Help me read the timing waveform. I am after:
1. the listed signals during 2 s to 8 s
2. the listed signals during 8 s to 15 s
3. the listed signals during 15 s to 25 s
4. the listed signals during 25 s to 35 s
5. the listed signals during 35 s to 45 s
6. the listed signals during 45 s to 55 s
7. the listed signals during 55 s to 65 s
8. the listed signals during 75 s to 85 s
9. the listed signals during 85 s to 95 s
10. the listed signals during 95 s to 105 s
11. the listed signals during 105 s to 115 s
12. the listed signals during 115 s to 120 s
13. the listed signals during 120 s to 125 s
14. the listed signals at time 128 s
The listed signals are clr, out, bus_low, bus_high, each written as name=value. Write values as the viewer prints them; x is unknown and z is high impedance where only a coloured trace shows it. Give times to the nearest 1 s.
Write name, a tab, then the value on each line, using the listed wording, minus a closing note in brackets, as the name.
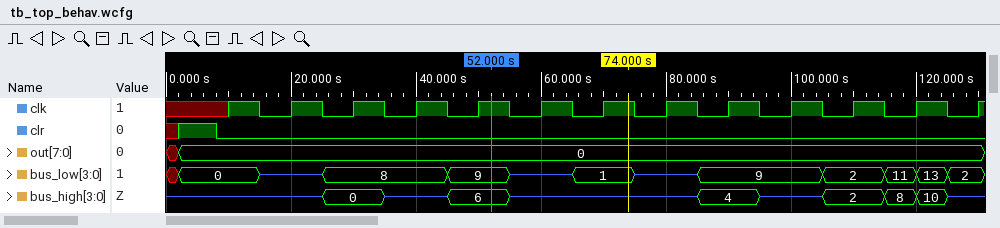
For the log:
the listed signals during 2 s to 8 s	clr=1, out=0, bus_low=0, bus_high=z
the listed signals during 8 s to 15 s	clr=0, out=0, bus_low=0, bus_high=z
the listed signals during 15 s to 25 s	clr=0, out=0, bus_low=z, bus_high=z
the listed signals during 25 s to 35 s	clr=0, out=0, bus_low=8, bus_high=0
the listed signals during 35 s to 45 s	clr=0, out=0, bus_low=8, bus_high=z
the listed signals during 45 s to 55 s	clr=0, out=0, bus_low=9, bus_high=6
the listed signals during 55 s to 65 s	clr=0, out=0, bus_low=z, bus_high=z
the listed signals during 75 s to 85 s	clr=0, out=0, bus_low=z, bus_high=z
the listed signals during 85 s to 95 s	clr=0, out=0, bus_low=9, bus_high=4
the listed signals during 95 s to 105 s	clr=0, out=0, bus_low=9, bus_high=z
the listed signals during 105 s to 115 s	clr=0, out=0, bus_low=2, bus_high=2
the listed signals during 115 s to 120 s	clr=0, out=0, bus_low=11, bus_high=8
the listed signals during 120 s to 125 s	clr=0, out=0, bus_low=13, bus_high=10
the listed signals at time 128 s	clr=0, out=0, bus_low=2, bus_high=z
